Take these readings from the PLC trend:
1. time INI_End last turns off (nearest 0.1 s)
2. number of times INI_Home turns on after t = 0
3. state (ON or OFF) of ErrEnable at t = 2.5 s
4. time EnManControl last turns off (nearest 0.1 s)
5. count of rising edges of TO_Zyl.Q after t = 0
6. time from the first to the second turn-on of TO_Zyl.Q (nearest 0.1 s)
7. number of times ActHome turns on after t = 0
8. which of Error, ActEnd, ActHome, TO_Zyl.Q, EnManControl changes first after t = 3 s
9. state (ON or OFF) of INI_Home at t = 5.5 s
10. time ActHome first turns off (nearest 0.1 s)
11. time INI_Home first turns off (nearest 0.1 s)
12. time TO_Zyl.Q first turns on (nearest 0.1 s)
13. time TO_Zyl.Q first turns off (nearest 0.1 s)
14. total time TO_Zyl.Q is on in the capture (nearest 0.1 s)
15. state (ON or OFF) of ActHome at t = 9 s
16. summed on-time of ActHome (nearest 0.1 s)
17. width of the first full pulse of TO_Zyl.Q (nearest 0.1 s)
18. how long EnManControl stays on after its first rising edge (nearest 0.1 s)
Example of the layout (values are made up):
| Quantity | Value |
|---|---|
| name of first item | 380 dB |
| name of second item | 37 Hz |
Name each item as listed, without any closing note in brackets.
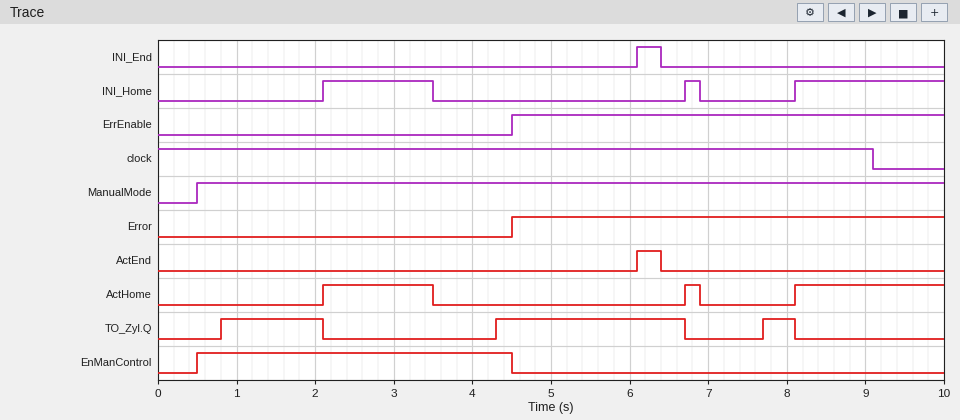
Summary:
| Quantity | Value |
|---|---|
| time INI_End last turns off | 6.4 s |
| number of times INI_Home turns on after t = 0 | 3 |
| state (ON or OFF) of ErrEnable at t = 2.5 s | OFF |
| time EnManControl last turns off | 4.5 s |
| count of rising edges of TO_Zyl.Q after t = 0 | 3 |
| time from the first to the second turn-on of TO_Zyl.Q | 3.5 s |
| number of times ActHome turns on after t = 0 | 3 |
| which of Error, ActEnd, ActHome, TO_Zyl.Q, EnManControl changes first after t = 3 s | ActHome |
| state (ON or OFF) of INI_Home at t = 5.5 s | OFF |
| time ActHome first turns off | 3.5 s |
| time INI_Home first turns off | 3.5 s |
| time TO_Zyl.Q first turns on | 0.8 s |
| time TO_Zyl.Q first turns off | 2.1 s |
| total time TO_Zyl.Q is on in the capture | 4.1 s |
| state (ON or OFF) of ActHome at t = 9 s | ON |
| summed on-time of ActHome | 3.5 s |
| width of the first full pulse of TO_Zyl.Q | 1.3 s |
| how long EnManControl stays on after its first rising edge | 4.0 s |
